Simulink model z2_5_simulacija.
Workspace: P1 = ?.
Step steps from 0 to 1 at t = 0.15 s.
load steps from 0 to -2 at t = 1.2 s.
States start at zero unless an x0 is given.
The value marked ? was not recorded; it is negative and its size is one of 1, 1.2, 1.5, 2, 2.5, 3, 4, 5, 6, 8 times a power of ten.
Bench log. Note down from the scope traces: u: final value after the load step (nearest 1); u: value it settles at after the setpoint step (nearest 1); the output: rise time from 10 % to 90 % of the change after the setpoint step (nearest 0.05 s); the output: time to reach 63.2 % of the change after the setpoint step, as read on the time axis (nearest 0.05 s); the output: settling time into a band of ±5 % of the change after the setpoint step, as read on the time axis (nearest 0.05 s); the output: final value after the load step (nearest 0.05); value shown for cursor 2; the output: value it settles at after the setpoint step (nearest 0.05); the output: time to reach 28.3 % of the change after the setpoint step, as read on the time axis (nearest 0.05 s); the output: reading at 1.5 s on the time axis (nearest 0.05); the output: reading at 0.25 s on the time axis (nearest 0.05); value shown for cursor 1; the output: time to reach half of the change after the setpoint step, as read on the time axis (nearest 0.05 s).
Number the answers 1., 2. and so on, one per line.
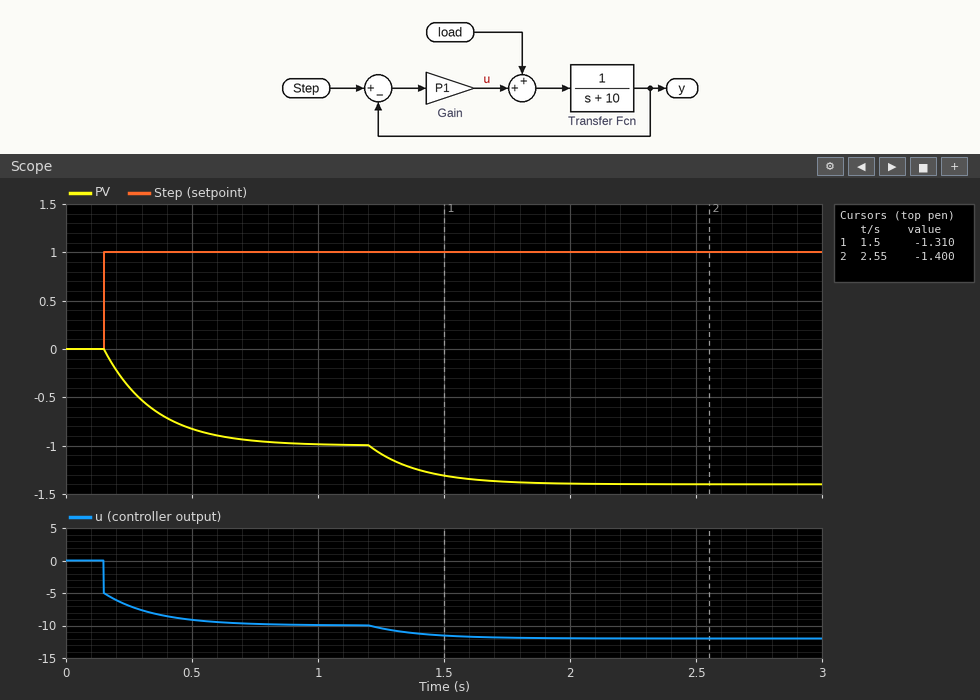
1. -12
2. -10
3. 0.45 s
4. 0.35 s
5. 0.75 s
6. -1.40
7. -1.400
8. -1.00
9. 0.20 s
10. -1.30
11. -0.40
12. -1.310
13. 0.30 s
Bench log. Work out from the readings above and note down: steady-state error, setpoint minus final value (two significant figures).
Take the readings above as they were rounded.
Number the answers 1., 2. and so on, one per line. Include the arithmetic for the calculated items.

1. 1 - (-1) = 2.0
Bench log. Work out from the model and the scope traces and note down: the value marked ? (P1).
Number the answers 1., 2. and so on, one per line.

1. -5
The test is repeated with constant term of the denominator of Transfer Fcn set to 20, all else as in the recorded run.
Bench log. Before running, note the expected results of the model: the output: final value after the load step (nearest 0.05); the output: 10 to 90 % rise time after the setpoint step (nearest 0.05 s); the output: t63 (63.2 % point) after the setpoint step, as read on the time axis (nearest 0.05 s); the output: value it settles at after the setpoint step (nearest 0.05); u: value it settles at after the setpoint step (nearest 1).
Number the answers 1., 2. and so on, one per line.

1. -0.45
2. 0.15 s
3. 0.20 s
4. -0.35
5. -7
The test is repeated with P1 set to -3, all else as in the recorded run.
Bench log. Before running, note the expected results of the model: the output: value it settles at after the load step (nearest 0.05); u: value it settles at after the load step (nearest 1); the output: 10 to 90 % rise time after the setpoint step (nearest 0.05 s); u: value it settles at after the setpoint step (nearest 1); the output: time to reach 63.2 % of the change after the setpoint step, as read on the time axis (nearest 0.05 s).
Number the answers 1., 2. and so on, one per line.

1. -0.70
2. -5
3. 0.30 s
4. -4
5. 0.30 s
